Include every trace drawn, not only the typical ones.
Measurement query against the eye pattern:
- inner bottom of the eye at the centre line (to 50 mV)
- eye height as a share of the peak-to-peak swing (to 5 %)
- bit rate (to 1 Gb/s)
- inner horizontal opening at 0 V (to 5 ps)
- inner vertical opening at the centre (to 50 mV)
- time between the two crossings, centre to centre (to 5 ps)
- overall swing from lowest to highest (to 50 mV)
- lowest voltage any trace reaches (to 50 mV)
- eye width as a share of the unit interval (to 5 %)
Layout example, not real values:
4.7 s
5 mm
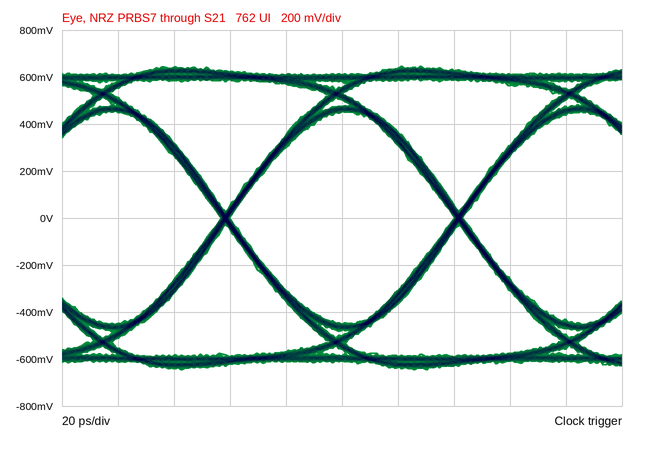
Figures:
-450 mV
70 %
12 Gb/s
80 ps
900 mV
85 ps
1.30 V
-650 mV
95 %
